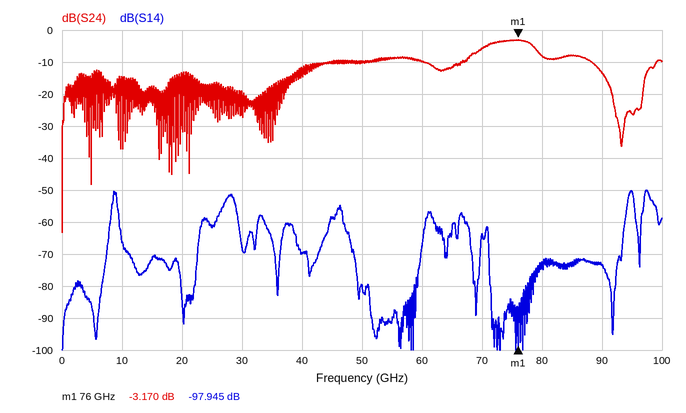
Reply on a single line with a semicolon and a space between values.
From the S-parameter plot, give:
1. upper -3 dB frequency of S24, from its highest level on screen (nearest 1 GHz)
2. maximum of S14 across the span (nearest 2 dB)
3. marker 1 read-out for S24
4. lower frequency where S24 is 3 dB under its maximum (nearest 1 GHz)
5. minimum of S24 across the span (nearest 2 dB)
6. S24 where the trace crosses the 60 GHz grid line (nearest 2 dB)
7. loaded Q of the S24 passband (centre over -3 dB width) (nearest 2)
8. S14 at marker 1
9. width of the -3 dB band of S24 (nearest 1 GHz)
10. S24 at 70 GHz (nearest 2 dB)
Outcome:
79 GHz; -50 dB; -3.170 dB; 70 GHz; -64 dB; -10 dB; 8; -97.945 dB; 9 GHz; -6 dB
